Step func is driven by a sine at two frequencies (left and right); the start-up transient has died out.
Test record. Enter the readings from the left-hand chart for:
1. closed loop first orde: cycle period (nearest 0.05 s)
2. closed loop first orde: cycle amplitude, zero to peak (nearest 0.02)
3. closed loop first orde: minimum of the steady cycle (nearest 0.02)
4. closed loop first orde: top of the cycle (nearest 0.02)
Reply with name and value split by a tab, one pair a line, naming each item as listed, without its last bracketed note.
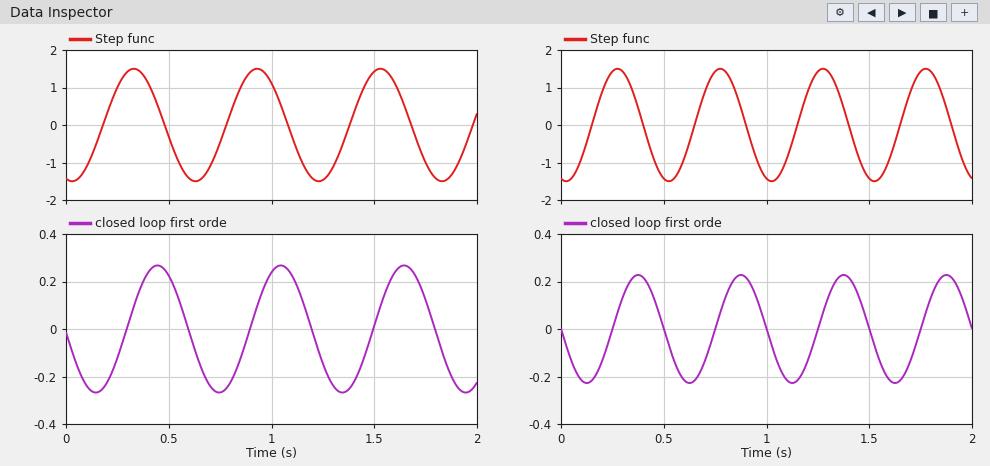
closed loop first orde: cycle period	0.60 s
closed loop first orde: cycle amplitude, zero to peak	0.26
closed loop first orde: minimum of the steady cycle	-0.26
closed loop first orde: top of the cycle	0.26
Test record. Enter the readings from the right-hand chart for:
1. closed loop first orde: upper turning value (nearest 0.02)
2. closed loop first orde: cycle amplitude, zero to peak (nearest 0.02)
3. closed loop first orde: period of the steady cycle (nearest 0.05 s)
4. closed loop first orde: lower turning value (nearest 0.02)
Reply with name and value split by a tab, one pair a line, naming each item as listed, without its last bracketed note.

closed loop first orde: upper turning value	0.22
closed loop first orde: cycle amplitude, zero to peak	0.22
closed loop first orde: period of the steady cycle	0.50 s
closed loop first orde: lower turning value	-0.22
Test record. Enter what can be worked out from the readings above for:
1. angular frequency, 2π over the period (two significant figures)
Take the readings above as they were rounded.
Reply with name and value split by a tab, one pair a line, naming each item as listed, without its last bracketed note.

angular frequency, 2π over the period	13 rad/s
